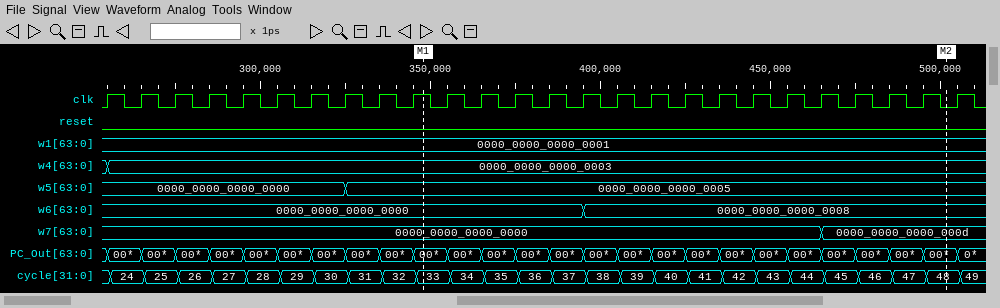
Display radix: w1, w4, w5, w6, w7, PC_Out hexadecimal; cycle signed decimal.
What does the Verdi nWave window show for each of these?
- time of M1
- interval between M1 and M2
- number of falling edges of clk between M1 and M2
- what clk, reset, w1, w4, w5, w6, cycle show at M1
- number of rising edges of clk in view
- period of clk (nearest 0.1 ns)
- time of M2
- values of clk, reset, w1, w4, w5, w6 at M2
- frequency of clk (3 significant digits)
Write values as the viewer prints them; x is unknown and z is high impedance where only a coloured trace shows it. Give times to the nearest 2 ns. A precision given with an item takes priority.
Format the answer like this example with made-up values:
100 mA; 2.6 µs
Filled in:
348 ns; 154 ns; 16; clk=1, reset=0, w1=0000_0000_0000_0001, w4=0000_0000_0000_0003, w5=0000_0000_0000_0005, w6=0000_0000_0000_0000, cycle=33; 26; 10 ns; 502 ns; clk=0, reset=0, w1=0000_0000_0000_0001, w4=0000_0000_0000_0003, w5=0000_0000_0000_0005, w6=0000_0000_0000_0008; 100 MHz
